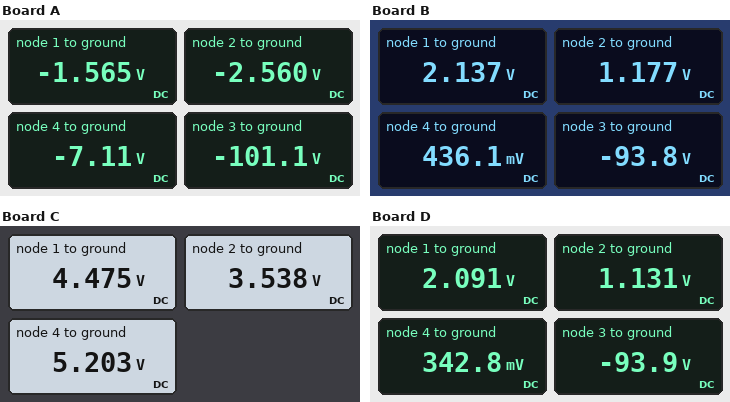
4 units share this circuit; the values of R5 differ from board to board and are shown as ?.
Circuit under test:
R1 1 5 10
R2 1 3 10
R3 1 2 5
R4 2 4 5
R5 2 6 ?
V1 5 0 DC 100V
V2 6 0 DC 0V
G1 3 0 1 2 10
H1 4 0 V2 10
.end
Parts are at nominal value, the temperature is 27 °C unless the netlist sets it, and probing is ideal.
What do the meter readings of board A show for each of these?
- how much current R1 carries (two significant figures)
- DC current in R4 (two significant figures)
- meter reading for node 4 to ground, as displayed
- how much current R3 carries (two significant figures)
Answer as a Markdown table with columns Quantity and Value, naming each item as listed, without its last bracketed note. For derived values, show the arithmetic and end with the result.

| Quantity | Value |
|---|---|
| how much current R1 carries | (100 V - (-1.565 V)) / 10 Ω = 10 A |
| DC current in R4 | (-2.56 V - (-7.11 V)) / 5 Ω = 910 mA |
| meter reading for node 4 to ground, as displayed | -7.11 V |
| how much current R3 carries | (-1.565 V - (-2.56 V)) / 5 Ω = 200 mA |
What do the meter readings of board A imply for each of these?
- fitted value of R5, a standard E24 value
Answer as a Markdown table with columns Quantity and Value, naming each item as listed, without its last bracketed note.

| Quantity | Value |
|---|---|
| fitted value of R5, a standard E24 value | 3.6 Ω |
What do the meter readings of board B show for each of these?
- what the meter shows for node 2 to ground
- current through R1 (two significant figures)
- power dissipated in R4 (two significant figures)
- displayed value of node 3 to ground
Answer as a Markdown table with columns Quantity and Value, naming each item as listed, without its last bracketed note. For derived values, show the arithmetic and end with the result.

| Quantity | Value |
|---|---|
| what the meter shows for node 2 to ground | 1.177 V |
| current through R1 | (100 V - 2.137 V) / 10 Ω = 9.8 A |
| power dissipated in R4 | (1.177 V - 436.1 mV)^2 / 5 Ω = 110 mW |
| displayed value of node 3 to ground | -93.8 V |
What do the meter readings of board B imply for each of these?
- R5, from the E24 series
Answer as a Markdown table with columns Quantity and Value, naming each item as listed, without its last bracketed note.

| Quantity | Value |
|---|---|
| R5, from the E24 series | 27 Ω |
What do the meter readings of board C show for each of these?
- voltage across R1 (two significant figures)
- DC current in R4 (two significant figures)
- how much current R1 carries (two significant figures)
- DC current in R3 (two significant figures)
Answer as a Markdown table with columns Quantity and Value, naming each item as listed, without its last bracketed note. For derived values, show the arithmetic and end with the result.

| Quantity | Value |
|---|---|
| voltage across R1 | 100 V - 4.475 V = 96 V |
| DC current in R4 | (5.203 V - 3.538 V) / 5 Ω = 330 mA |
| how much current R1 carries | (100 V - 4.475 V) / 10 Ω = 9.6 A |
| DC current in R3 | (4.475 V - 3.538 V) / 5 Ω = 190 mA |
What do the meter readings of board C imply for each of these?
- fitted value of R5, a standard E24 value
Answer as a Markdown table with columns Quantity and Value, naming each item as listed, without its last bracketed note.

| Quantity | Value |
|---|---|
| fitted value of R5, a standard E24 value | 6.8 Ω |
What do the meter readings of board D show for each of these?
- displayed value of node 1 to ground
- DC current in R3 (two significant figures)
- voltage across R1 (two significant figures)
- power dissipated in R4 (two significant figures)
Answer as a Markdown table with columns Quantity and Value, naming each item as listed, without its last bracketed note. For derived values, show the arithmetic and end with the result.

| Quantity | Value |
|---|---|
| displayed value of node 1 to ground | 2.091 V |
| DC current in R3 | (2.091 V - 1.131 V) / 5 Ω = 190 mA |
| voltage across R1 | 100 V - 2.091 V = 98 V |
| power dissipated in R4 | (1.131 V - 342.8 mV)^2 / 5 Ω = 120 mW |
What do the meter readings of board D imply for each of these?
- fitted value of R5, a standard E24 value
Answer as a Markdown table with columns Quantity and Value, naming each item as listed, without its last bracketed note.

| Quantity | Value |
|---|---|
| fitted value of R5, a standard E24 value | 33 Ω |
